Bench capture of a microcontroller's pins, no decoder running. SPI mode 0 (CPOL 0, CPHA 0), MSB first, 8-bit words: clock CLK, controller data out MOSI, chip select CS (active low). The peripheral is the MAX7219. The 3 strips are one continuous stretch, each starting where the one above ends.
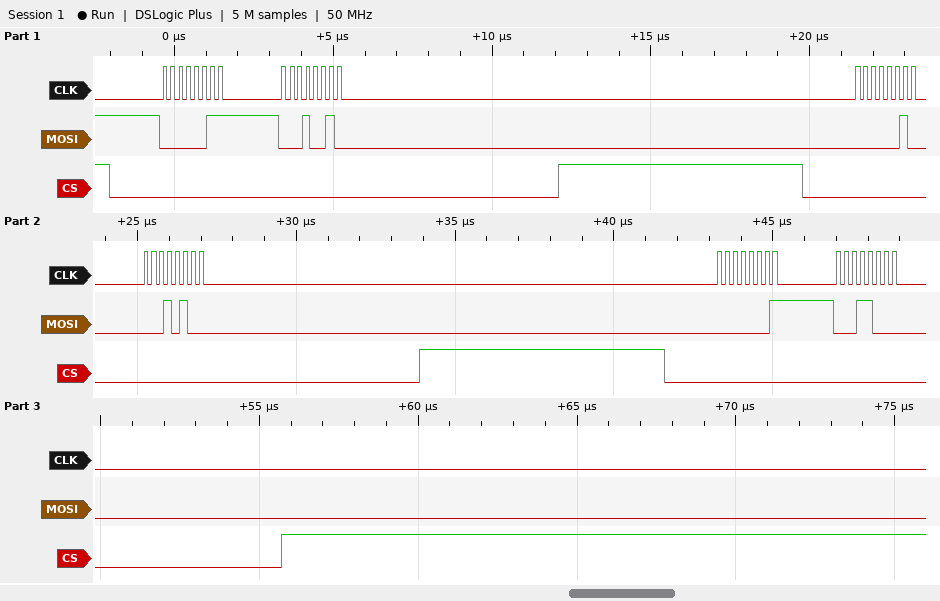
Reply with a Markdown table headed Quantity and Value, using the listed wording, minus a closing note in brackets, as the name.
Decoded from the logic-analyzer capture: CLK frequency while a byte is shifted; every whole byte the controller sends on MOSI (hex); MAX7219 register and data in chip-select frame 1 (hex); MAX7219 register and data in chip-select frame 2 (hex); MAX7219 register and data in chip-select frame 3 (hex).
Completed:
| Quantity | Value |
|---|---|
| CLK frequency while a byte is shifted | 4 MHz |
| every whole byte the controller sends on MOSI | 03 12 02 14 01 18 |
| MAX7219 register and data in chip-select frame 1 | register 0x3, data 0x12 |
| MAX7219 register and data in chip-select frame 2 | register 0x2, data 0x14 |
| MAX7219 register and data in chip-select frame 3 | register 0x1, data 0x18 |
